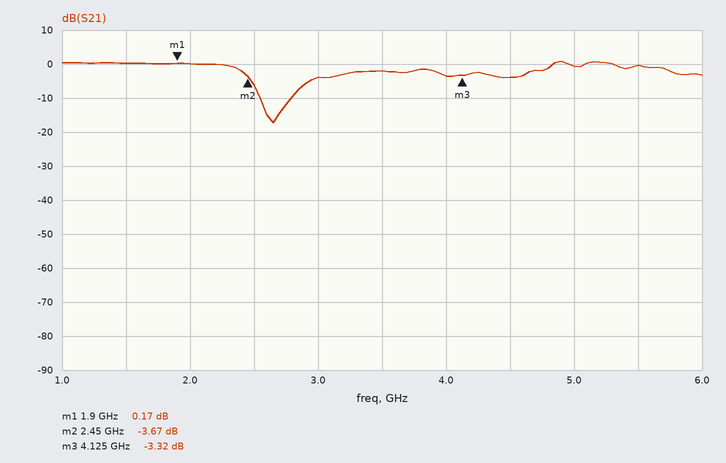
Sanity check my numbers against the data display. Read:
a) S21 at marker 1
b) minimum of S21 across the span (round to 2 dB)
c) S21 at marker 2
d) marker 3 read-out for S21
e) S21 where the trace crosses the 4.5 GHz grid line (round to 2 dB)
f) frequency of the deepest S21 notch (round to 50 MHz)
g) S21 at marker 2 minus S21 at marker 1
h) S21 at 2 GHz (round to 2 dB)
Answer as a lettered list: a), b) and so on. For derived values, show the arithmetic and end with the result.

a) 0.17 dB
b) -18 dB
c) -3.67 dB
d) -3.32 dB
e) -4 dB
f) 2.65 GHz
g) -3.67 − (0.17) = -3.84 dB
h) 0 dB
